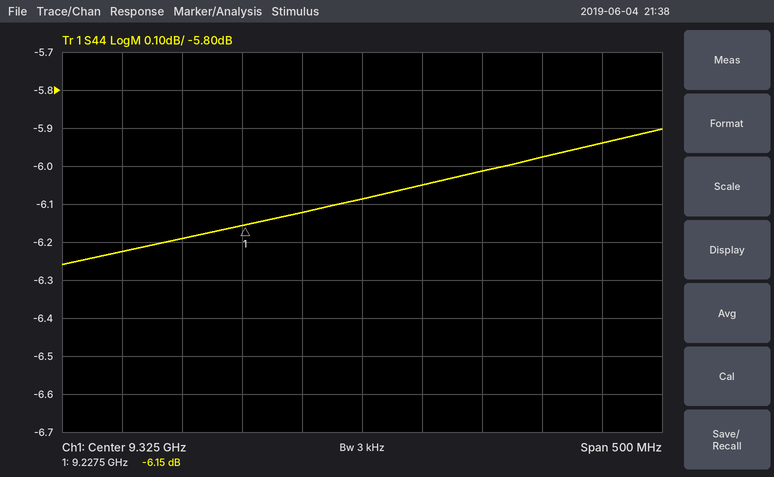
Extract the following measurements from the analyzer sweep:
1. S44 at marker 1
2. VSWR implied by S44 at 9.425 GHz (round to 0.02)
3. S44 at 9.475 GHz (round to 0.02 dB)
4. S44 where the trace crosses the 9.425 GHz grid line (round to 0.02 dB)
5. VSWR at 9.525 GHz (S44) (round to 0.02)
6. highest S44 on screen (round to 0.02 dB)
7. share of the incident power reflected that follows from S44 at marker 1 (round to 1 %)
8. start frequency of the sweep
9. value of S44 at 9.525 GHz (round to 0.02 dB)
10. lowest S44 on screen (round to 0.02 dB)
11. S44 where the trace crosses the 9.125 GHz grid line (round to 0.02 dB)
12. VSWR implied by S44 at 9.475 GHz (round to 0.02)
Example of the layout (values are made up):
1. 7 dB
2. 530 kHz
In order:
1. -6.15 dB
2. 3.00
3. -5.98 dB
4. -6.02 dB
5. 3.04
6. -5.90 dB
7. 24 %
8. 9.075 GHz
9. -5.94 dB
10. -6.26 dB
11. -6.22 dB
12. 3.02
